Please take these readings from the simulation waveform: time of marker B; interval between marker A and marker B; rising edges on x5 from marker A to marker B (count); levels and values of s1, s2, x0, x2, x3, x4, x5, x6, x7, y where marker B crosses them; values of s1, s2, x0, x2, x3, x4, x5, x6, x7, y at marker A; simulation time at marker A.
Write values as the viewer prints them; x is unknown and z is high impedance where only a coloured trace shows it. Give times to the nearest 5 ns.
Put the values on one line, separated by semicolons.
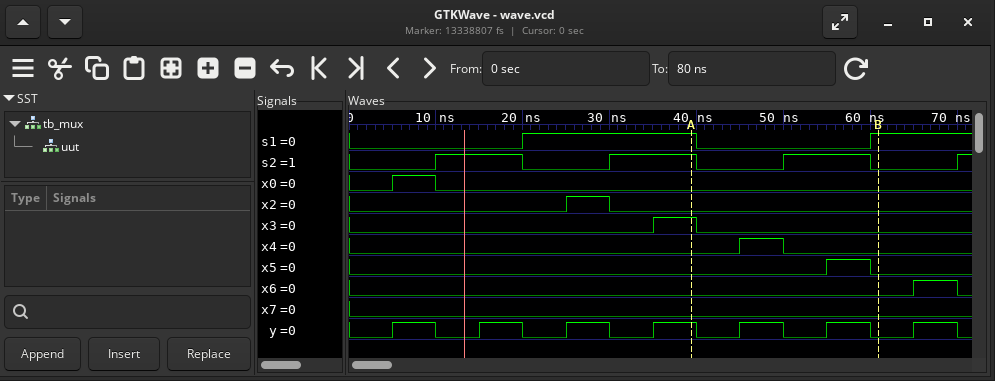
60 ns; 20 ns; 1; s1=1, s2=0, x0=0, x2=0, x3=0, x4=0, x5=0, x6=0, x7=0, y=0; s1=1, s2=1, x0=0, x2=0, x3=1, x4=0, x5=0, x6=0, x7=0, y=1; 40 ns
